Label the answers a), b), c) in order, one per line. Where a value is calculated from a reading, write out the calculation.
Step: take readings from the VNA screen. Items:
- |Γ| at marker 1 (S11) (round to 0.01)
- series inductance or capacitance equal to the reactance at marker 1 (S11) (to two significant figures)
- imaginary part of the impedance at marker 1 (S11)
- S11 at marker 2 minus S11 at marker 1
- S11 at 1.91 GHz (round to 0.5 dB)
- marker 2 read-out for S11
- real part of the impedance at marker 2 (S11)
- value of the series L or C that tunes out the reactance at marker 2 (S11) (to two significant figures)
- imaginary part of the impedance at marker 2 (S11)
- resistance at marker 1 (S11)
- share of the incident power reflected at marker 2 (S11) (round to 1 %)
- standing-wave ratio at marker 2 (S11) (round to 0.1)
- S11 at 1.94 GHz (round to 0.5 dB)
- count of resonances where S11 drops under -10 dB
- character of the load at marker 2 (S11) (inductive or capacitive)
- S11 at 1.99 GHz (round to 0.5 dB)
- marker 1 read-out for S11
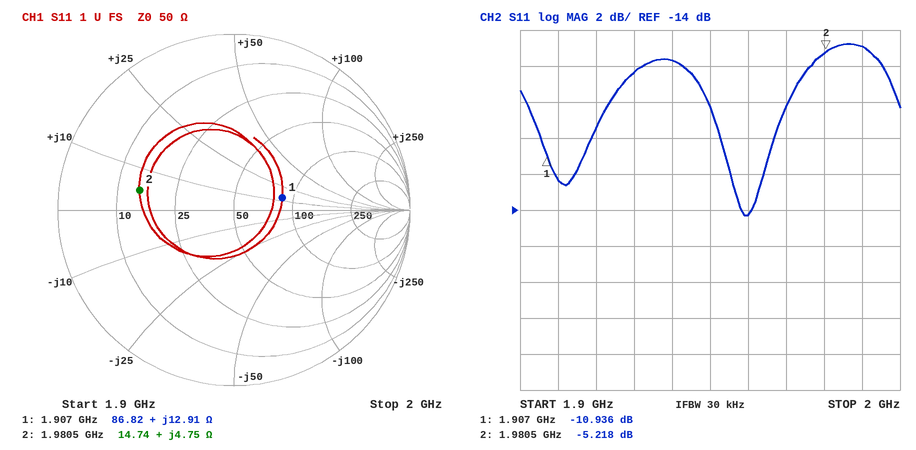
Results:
a) 0.28
b) L = 12.91 Ω/(2π × 1.907 GHz) ≈ 1.1 nH
c) +12.91 Ω
d) -5.218 − (-10.936) = 5.718 dB
e) -12.5 dB
f) -5.218 dB
g) 14.74 Ω
h) C = 1/(2π × 1.9805 GHz × 4.75 Ω) ≈ 17 pF
i) +4.75 Ω
j) 86.82 Ω
k) 10^(-5.218/10) ≈ 30 %
l) 3.4
m) -5.5 dB
n) 2
o) inductive
p) -5.0 dB
q) -10.936 dB
